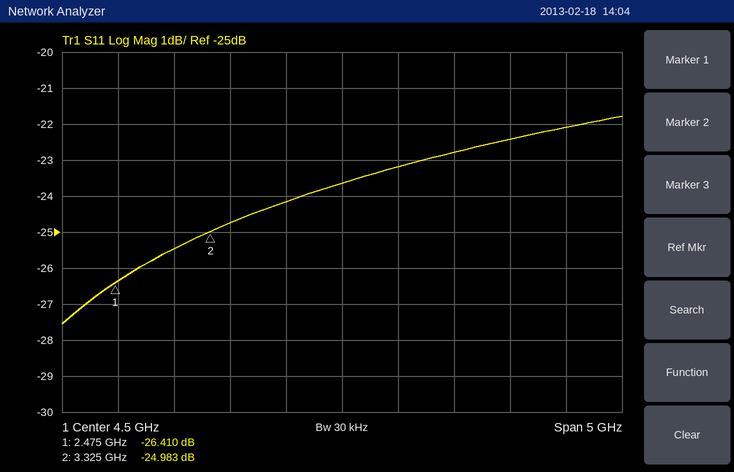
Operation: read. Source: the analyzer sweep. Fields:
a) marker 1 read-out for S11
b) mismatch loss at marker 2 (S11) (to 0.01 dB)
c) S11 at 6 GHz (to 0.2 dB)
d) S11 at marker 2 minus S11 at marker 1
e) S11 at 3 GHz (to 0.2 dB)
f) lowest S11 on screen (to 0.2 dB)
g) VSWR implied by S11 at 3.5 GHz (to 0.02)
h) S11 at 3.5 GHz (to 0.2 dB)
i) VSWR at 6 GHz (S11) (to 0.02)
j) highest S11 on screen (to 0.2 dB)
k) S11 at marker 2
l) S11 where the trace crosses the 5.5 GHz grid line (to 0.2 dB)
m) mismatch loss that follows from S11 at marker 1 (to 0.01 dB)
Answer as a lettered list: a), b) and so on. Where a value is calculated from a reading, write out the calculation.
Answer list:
a) -26.410 dB
b) −10 log10(1 − 10^(-24.983/10)) ≈ 0.01 dB
c) -22.4 dB
d) -24.983 − (-26.41) = 1.427 dB
e) -25.4 dB
f) -27.6 dB
g) |Γ| = 10^(-24.8/20) = 0.0575; VSWR = (1 + 0.0575)/(1 − 0.0575) ≈ 1.12
h) -24.8 dB
i) |Γ| = 10^(-22.4/20) = 0.0759; VSWR = (1 + 0.0759)/(1 − 0.0759) ≈ 1.16
j) -21.8 dB
k) -24.983 dB
l) -22.8 dB
m) −10 log10(1 − 10^(-26.41/10)) ≈ 0.01 dB
